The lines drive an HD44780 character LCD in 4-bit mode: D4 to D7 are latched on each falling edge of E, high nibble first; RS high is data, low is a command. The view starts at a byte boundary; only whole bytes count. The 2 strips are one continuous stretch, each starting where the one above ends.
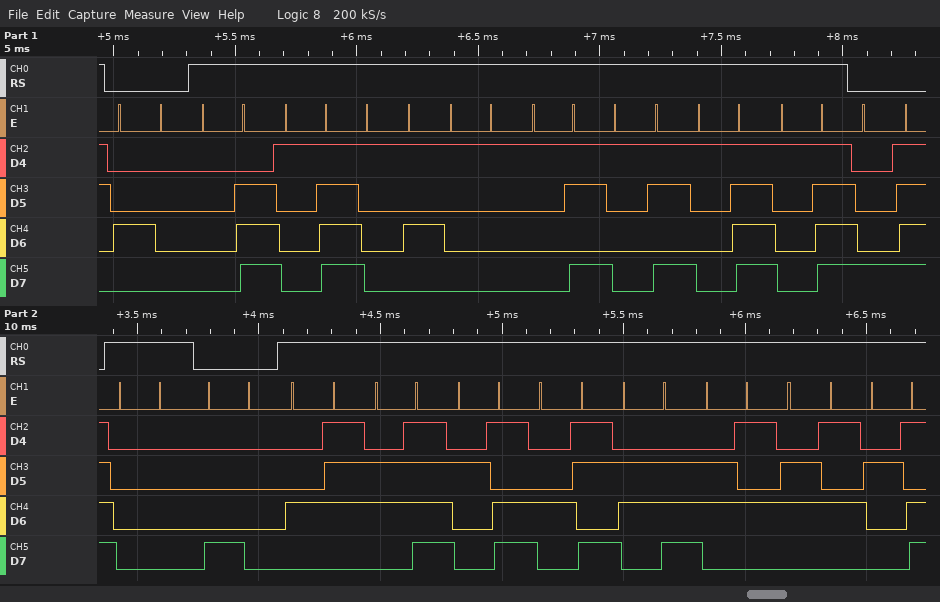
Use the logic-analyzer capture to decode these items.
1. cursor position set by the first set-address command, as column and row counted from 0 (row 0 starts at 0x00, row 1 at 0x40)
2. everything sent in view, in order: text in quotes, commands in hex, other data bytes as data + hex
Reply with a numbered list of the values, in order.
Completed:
1. column 15, row 0
2. 0x40 data 0E 1F 15 11 1B 1B 1F 1F 0x8F data 00 0x80 "Go-Knee-"
